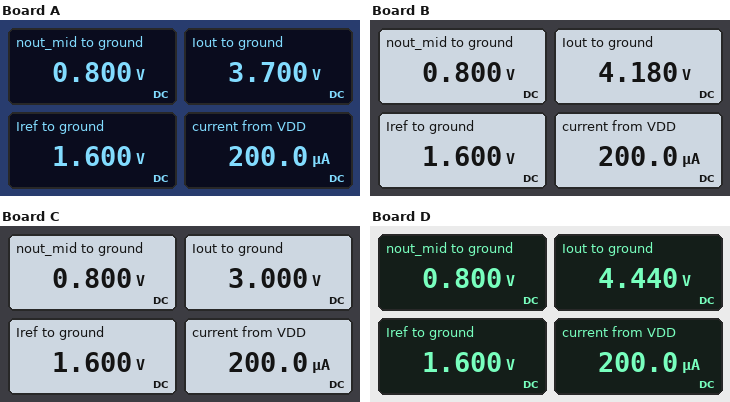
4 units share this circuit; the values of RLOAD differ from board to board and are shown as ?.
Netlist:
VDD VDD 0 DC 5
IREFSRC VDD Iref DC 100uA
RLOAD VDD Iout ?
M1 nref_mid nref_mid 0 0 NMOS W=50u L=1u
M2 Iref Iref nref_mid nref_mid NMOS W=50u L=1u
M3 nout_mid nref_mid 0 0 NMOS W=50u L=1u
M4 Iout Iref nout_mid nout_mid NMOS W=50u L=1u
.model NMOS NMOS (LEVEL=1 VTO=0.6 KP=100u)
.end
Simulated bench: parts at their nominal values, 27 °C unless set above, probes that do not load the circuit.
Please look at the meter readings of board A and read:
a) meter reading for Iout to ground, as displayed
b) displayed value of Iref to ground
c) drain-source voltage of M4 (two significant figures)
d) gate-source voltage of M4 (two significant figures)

3.700 V
1.600 V
2.9 V
800 mV
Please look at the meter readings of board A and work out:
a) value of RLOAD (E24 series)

13 kΩ
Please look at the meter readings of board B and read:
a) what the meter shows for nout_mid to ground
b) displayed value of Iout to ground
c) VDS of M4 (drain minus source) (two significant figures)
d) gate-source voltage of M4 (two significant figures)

0.800 V
4.180 V
3.4 V
800 mV
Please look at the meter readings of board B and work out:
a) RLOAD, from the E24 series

8.2 kΩ
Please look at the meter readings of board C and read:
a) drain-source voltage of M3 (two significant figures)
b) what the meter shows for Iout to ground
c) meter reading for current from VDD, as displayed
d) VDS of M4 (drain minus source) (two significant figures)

800 mV
3.000 V
200.0 µA
2.2 V
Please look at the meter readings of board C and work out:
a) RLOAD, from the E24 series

20 kΩ
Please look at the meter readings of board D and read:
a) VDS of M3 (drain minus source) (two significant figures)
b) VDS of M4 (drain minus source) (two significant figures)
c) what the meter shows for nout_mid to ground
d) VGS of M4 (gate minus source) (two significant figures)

800 mV
3.6 V
0.800 V
800 mV
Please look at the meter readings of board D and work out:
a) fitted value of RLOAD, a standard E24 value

5.6 kΩ
